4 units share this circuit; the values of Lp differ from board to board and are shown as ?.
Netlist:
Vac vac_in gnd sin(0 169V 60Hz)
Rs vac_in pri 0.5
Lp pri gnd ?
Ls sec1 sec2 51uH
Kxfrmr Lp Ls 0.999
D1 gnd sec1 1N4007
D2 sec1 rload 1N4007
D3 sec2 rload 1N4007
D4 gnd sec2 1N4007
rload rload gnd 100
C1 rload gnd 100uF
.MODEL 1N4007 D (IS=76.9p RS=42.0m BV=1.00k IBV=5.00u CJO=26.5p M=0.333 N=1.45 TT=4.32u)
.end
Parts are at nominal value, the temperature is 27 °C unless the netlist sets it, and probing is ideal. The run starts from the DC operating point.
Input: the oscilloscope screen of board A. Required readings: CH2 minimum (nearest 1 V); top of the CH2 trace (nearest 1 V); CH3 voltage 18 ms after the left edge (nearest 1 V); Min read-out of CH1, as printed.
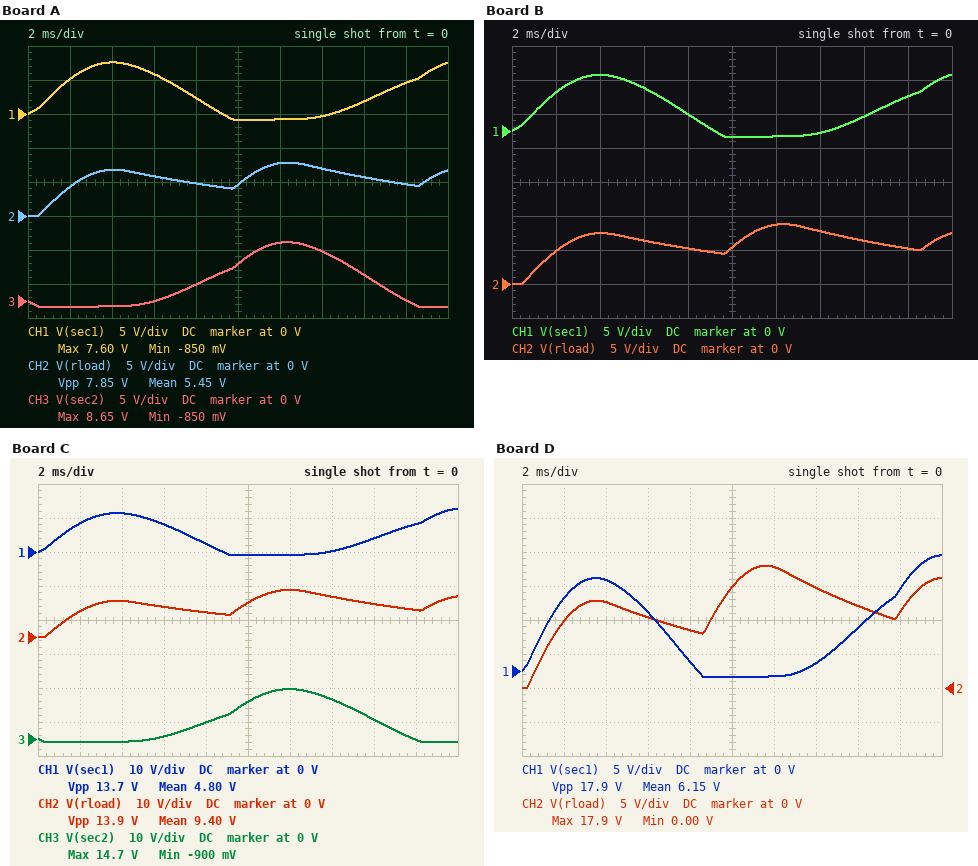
0 V
8 V
0 V
-850 mV
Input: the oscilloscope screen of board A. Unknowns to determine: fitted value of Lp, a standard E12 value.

18 mH
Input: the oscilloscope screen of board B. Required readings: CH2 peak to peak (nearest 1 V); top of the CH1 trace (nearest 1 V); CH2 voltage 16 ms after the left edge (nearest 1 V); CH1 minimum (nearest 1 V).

9 V
8 V
6 V
-1 V
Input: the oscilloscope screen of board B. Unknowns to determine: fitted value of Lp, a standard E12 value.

15 mH
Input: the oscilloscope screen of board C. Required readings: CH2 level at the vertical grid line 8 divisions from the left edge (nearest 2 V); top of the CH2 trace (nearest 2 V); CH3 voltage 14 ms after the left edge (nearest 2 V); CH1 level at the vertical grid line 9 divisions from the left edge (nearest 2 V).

10 V
14 V
12 V
8 V
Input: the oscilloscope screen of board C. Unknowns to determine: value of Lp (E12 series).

6.8 mH
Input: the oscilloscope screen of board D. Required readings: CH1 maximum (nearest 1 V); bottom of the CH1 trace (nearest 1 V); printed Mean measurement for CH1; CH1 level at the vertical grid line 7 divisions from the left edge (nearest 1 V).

17 V
-1 V
6.15 V
1 V
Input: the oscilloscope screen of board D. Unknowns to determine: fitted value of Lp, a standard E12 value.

3.9 mH
